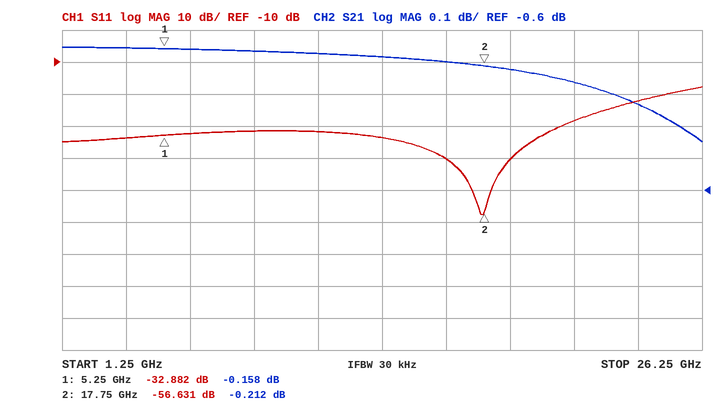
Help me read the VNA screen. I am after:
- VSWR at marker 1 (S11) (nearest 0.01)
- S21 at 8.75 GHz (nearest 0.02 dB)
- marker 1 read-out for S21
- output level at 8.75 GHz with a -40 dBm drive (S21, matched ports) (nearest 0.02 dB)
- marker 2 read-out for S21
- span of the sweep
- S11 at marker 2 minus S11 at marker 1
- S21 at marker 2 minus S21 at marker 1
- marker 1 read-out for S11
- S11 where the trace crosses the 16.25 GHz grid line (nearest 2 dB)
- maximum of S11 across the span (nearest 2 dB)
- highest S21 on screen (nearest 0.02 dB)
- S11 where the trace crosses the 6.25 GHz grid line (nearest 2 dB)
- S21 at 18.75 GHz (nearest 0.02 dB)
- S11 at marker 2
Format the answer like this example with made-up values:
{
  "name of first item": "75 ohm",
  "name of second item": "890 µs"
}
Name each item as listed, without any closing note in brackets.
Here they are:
{
  "VSWR at marker 1 (S11)": "1.05",
  "S21 at 8.75 GHz": "-0.16 dB",
  "marker 1 read-out for S21": "-0.158 dB",
  "output level at 8.75 GHz with a -40 dBm drive (S21, matched ports)": "-40.16 dBm",
  "marker 2 read-out for S21": "-0.212 dB",
  "span of the sweep": "25 GHz",
  "S11 at marker 2 minus S11 at marker 1": "-23.749 dB",
  "S21 at marker 2 minus S21 at marker 1": "-0.054 dB",
  "marker 1 read-out for S11": "-32.882 dB",
  "S11 where the trace crosses the 16.25 GHz grid line": "-40 dB",
  "maximum of S11 across the span": "-18 dB",
  "highest S21 on screen": "-0.16 dB",
  "S11 where the trace crosses the 6.25 GHz grid line": "-32 dB",
  "S21 at 18.75 GHz": "-0.22 dB",
  "S11 at marker 2": "-56.631 dB"
}
